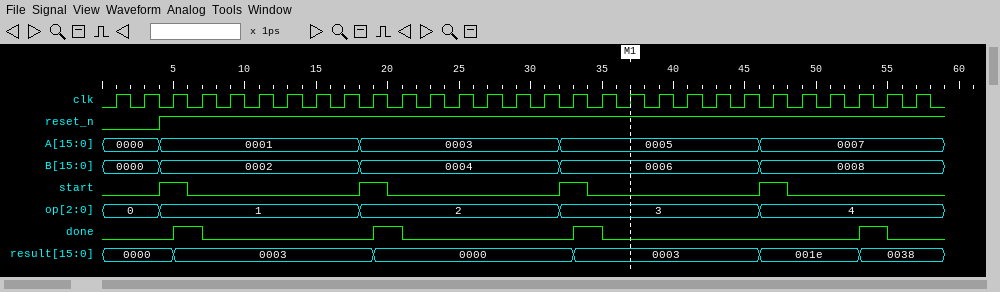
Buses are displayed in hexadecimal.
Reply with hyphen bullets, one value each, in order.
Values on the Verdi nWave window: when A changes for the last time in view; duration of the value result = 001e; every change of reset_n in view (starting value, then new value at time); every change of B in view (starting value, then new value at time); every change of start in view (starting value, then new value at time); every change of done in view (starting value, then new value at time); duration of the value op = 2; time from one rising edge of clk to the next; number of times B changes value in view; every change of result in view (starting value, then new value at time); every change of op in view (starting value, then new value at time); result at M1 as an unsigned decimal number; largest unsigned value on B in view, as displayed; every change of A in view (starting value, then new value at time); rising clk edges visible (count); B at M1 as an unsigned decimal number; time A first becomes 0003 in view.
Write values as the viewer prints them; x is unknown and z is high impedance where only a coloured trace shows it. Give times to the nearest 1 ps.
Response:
- 46 ps
- 7 ps
- 0, 1 at 4 ps
- 0000, 0002 at 4 ps, 0004 at 18 ps, 0006 at 32 ps, 0008 at 46 ps
- 0, 1 at 4 ps, 0 at 6 ps, 1 at 18 ps, 0 at 20 ps, 1 at 32 ps, 0 at 34 ps, 1 at 46 ps, 0 at 48 ps
- 0, 1 at 5 ps, 0 at 7 ps, 1 at 19 ps, 0 at 21 ps, 1 at 33 ps, 0 at 35 ps, 1 at 53 ps, 0 at 55 ps
- 14 ps
- 2 ps
- 4
- 0000, 0003 at 5 ps, 0000 at 19 ps, 0003 at 33 ps, 001e at 46 ps, 0038 at 53 ps
- 0, 1 at 4 ps, 2 at 18 ps, 3 at 32 ps, 4 at 46 ps
- 3
- 0008
- 0000, 0001 at 4 ps, 0003 at 18 ps, 0005 at 32 ps, 0007 at 46 ps
- 29
- 6
- 18 ps
